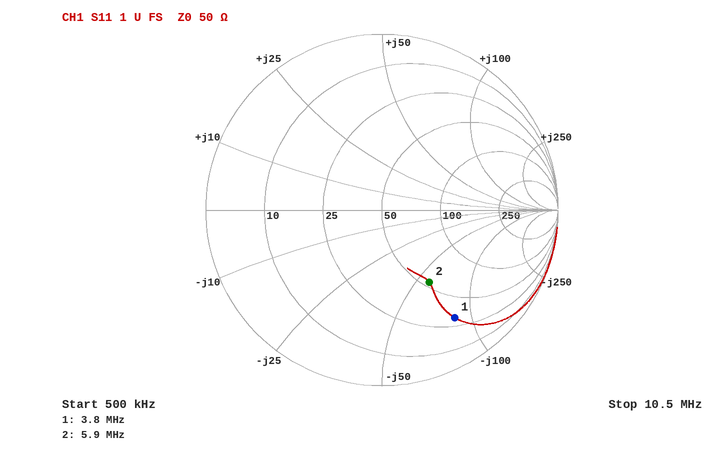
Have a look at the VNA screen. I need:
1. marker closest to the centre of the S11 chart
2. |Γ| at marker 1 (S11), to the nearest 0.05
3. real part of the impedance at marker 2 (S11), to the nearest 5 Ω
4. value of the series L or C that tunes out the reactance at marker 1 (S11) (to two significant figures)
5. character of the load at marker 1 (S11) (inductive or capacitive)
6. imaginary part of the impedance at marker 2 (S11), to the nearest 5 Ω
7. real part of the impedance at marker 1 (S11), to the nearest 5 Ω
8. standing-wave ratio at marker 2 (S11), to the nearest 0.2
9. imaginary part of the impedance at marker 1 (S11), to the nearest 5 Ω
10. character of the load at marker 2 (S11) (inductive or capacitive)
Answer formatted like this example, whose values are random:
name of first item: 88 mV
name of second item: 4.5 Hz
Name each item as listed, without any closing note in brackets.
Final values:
marker closest to the centre of the S11 chart: marker 2
|Γ| at marker 1 (S11), to the nearest 0.05: 0.75
real part of the impedance at marker 2 (S11), to the nearest 5 Ω: 55 Ω
value of the series L or C that tunes out the reactance at marker 1 (S11): 3.6 µH
character of the load at marker 1 (S11): capacitive
imaginary part of the impedance at marker 2 (S11), to the nearest 5 Ω: -60 Ω
real part of the impedance at marker 1 (S11), to the nearest 5 Ω: 30 Ω
standing-wave ratio at marker 2 (S11), to the nearest 0.2: 3.0
imaginary part of the impedance at marker 1 (S11), to the nearest 5 Ω: -85 Ω
character of the load at marker 2 (S11): capacitive
